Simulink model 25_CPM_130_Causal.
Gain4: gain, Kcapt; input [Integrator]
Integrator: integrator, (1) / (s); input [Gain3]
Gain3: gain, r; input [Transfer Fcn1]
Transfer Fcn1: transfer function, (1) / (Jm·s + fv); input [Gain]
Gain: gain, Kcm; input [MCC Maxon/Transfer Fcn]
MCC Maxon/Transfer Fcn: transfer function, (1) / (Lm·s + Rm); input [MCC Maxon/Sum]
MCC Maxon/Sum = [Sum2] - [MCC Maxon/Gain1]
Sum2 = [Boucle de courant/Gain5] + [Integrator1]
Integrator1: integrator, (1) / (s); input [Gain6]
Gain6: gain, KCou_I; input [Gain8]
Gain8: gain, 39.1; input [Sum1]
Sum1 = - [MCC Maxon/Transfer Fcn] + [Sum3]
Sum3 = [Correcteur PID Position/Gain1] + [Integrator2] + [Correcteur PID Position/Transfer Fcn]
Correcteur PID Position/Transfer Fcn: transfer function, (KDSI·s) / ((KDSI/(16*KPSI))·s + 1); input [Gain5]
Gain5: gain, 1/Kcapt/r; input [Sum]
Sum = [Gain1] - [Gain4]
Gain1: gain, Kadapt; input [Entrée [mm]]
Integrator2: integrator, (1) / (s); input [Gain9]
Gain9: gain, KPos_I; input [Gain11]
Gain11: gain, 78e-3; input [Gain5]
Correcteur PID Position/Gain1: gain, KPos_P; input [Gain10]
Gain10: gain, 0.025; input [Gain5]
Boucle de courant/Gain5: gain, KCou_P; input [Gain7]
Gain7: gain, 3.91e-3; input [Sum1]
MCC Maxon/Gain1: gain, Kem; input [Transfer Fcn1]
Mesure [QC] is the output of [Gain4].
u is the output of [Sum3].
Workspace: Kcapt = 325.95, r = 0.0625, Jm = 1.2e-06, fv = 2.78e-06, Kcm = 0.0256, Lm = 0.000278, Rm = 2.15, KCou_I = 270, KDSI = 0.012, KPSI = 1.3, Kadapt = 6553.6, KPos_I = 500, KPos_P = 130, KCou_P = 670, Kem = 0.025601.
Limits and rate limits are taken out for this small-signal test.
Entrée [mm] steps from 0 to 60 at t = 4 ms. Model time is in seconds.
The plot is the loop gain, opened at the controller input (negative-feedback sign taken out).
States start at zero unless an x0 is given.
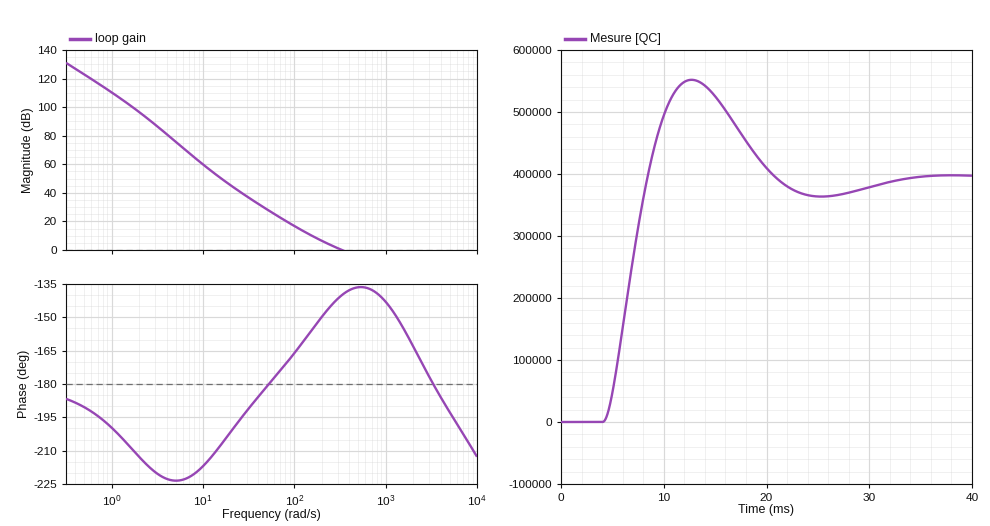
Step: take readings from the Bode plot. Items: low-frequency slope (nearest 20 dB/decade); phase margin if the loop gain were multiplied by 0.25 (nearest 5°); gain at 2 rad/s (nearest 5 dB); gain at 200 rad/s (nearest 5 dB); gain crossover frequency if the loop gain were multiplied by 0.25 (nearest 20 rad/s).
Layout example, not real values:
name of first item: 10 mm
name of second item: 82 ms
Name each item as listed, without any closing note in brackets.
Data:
low-frequency slope: -40 dB/decade
phase margin if the loop gain were multiplied by 0.25: 20°
gain at 2 rad/s: 95 dB
gain at 200 rad/s: 5 dB
gain crossover frequency if the loop gain were multiplied by 0.25: 140 rad/s
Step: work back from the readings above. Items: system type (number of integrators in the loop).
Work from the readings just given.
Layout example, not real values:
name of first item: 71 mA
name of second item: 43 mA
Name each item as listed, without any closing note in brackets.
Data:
system type: 2
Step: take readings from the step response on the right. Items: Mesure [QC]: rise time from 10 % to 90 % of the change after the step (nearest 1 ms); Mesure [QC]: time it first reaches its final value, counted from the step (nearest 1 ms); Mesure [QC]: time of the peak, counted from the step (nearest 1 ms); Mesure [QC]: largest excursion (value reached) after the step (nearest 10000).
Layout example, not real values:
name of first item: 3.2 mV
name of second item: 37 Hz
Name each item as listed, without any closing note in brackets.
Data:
Mesure [QC]: rise time from 10 % to 90 % of the change after the step: 3 ms
Mesure [QC]: time it first reaches its final value, counted from the step: 4 ms
Mesure [QC]: time of the peak, counted from the step: 9 ms
Mesure [QC]: largest excursion (value reached) after the step: 550000
